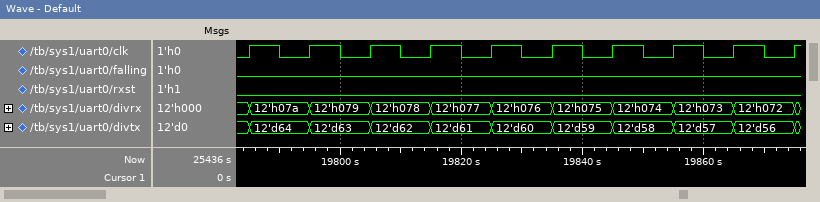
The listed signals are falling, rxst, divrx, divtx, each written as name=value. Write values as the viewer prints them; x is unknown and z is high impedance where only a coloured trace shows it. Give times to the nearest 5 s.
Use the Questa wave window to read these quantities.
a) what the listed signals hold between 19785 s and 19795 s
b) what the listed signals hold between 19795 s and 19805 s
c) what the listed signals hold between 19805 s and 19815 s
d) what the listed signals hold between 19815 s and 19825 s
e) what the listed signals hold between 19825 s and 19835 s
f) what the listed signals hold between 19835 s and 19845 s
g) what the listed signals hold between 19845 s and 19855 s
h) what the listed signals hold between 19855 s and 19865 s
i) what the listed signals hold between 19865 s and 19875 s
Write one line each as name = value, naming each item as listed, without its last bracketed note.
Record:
what the listed signals hold between 19785 s and 19795 s = falling=0, rxst=0, divrx=12'h07a, divtx=12'd64
what the listed signals hold between 19795 s and 19805 s = falling=0, rxst=0, divrx=12'h079, divtx=12'd63
what the listed signals hold between 19805 s and 19815 s = falling=0, rxst=0, divrx=12'h078, divtx=12'd62
what the listed signals hold between 19815 s and 19825 s = falling=0, rxst=0, divrx=12'h077, divtx=12'd61
what the listed signals hold between 19825 s and 19835 s = falling=0, rxst=0, divrx=12'h076, divtx=12'd60
what the listed signals hold between 19835 s and 19845 s = falling=0, rxst=0, divrx=12'h075, divtx=12'd59
what the listed signals hold between 19845 s and 19855 s = falling=0, rxst=0, divrx=12'h074, divtx=12'd58
what the listed signals hold between 19855 s and 19865 s = falling=0, rxst=0, divrx=12'h073, divtx=12'd57
what the listed signals hold between 19865 s and 19875 s = falling=0, rxst=0, divrx=12'h072, divtx=12'd56
